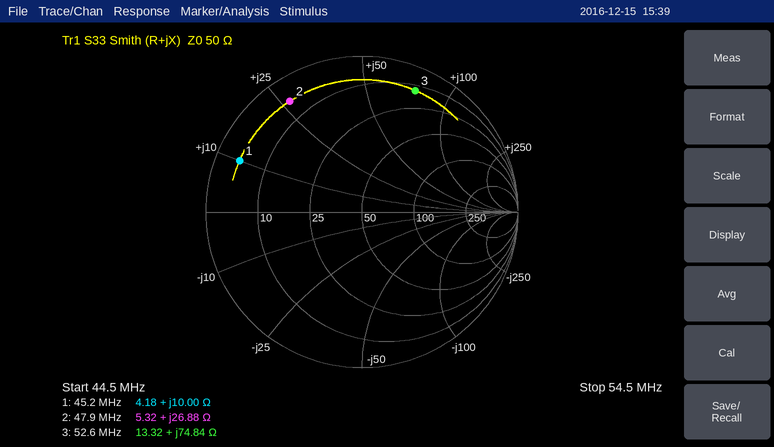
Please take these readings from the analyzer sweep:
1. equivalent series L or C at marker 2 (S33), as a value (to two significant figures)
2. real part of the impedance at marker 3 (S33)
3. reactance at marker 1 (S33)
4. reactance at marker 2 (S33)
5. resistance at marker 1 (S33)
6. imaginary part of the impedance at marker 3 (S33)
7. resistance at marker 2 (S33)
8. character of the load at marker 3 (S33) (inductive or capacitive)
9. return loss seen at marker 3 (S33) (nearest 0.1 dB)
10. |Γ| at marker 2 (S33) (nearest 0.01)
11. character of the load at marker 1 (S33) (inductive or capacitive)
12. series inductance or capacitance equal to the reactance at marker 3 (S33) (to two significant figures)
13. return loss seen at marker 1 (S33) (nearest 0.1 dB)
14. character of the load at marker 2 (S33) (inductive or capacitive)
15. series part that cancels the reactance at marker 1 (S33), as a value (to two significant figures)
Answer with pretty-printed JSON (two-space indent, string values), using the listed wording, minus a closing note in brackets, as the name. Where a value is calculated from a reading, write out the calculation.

{
  "equivalent series L or C at marker 2 (S33), as a value": "L = 26.88 Ω/(2π × 47.9 MHz) ≈ 89 nH",
  "real part of the impedance at marker 3": "13.32 Ω",
  "reactance at marker 1": "+10.00 Ω",
  "reactance at marker 2": "+26.88 Ω",
  "resistance at marker 1": "4.18 Ω",
  "imaginary part of the impedance at marker 3": "+74.84 Ω",
  "resistance at marker 2": "5.32 Ω",
  "character of the load at marker 3 (S33)": "inductive",
  "return loss seen at marker 3 (S33)": "1.4 dB",
  "|Γ| at marker 2 (S33)": "0.85",
  "character of the load at marker 1 (S33)": "inductive",
  "series inductance or capacitance equal to the reactance at marker 3 (S33)": "L = 74.84 Ω/(2π × 52.6 MHz) ≈ 226 nH, so 230 nH to two significant figures",
  "return loss seen at marker 1 (S33)": "1.4 dB",
  "character of the load at marker 2 (S33)": "inductive",
  "series part that cancels the reactance at marker 1 (S33), as a value": "C = 1/(2π × 45.2 MHz × 10 Ω) ≈ 352 pF, so 350 pF to two significant figures"
}
